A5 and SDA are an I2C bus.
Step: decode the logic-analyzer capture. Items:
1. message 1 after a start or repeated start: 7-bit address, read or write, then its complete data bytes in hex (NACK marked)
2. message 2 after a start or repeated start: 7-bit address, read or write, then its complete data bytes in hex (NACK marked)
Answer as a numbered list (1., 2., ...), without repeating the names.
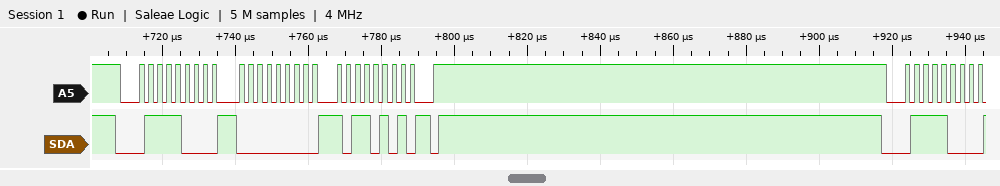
1. 0x3C write: 00 B5
2. 0x3C write
